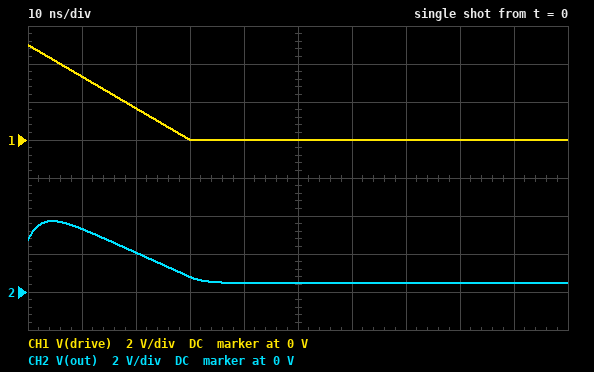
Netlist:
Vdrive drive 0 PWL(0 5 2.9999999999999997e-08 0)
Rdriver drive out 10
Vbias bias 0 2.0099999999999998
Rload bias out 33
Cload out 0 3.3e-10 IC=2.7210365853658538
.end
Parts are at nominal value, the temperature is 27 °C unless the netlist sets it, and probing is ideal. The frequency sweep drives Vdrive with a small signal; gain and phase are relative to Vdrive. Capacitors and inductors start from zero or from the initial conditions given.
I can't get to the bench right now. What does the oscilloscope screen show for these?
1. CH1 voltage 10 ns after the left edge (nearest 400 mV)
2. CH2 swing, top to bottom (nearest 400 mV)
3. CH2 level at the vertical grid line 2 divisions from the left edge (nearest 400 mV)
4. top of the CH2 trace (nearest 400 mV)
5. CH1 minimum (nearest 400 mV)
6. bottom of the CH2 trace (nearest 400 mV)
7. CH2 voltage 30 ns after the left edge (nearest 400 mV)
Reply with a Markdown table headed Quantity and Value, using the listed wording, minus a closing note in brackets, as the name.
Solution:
| Quantity | Value |
|---|---|
| CH1 voltage 10 ns after the left edge | 3.2 V |
| CH2 swing, top to bottom | 3.2 V |
| CH2 level at the vertical grid line 2 divisions from the left edge | 2.0 V |
| top of the CH2 trace | 3.6 V |
| CH1 minimum | 0 V |
| bottom of the CH2 trace | 400 mV |
| CH2 voltage 30 ns after the left edge | 800 mV |
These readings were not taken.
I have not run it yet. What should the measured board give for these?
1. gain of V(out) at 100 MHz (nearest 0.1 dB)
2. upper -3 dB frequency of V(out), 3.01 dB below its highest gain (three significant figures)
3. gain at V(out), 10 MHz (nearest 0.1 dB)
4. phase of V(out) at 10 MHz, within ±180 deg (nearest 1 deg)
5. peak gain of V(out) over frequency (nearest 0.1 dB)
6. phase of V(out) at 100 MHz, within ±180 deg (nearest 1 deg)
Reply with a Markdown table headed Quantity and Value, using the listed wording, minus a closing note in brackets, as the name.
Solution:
| Quantity | Value |
|---|---|
| gain of V(out) at 100 MHz | -7.8 dB |
| upper -3 dB frequency of V(out), 3.01 dB below its highest gain | 62.8 MHz |
| gain at V(out), 10 MHz | -2.4 dB |
| phase of V(out) at 10 MHz, within ±180 deg | -9 deg |
| peak gain of V(out) over frequency | -2.3 dB |
| phase of V(out) at 100 MHz, within ±180 deg | -58 deg |
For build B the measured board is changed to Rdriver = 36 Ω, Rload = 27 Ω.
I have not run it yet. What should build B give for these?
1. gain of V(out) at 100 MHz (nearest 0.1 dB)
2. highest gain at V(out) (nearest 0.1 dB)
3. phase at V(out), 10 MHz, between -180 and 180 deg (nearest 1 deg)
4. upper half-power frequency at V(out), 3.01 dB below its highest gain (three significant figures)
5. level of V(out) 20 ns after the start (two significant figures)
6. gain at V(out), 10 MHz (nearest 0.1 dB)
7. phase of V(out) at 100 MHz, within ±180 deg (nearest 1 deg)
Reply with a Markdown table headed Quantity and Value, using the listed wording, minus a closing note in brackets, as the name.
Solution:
| Quantity | Value |
|---|---|
| gain of V(out) at 100 MHz | -17.9 dB |
| highest gain at V(out) | -7.4 dB |
| phase at V(out), 10 MHz, between -180 and 180 deg | -18 deg |
| upper half-power frequency at V(out), 3.01 dB below its highest gain | 31.3 MHz |
| level of V(out) 20 ns after the start | 2.2 V |
| gain at V(out), 10 MHz | -7.8 dB |
| phase of V(out) at 100 MHz, within ±180 deg | -73 deg |
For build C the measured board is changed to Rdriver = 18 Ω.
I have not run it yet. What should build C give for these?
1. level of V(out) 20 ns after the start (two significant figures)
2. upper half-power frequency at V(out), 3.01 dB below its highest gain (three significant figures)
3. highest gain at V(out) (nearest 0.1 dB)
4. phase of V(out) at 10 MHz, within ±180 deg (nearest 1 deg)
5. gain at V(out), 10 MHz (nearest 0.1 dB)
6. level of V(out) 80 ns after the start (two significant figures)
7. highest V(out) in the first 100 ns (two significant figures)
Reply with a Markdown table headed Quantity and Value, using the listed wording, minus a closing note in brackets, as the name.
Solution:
| Quantity | Value |
|---|---|
| level of V(out) 20 ns after the start | 2.2 V |
| upper half-power frequency at V(out), 3.01 dB below its highest gain | 41.4 MHz |
| highest gain at V(out) | -3.8 dB |
| phase of V(out) at 10 MHz, within ±180 deg | -14 deg |
| gain at V(out), 10 MHz | -4.0 dB |
| level of V(out) 80 ns after the start | 710 mV |
| highest V(out) in the first 100 ns | 3.4 V |
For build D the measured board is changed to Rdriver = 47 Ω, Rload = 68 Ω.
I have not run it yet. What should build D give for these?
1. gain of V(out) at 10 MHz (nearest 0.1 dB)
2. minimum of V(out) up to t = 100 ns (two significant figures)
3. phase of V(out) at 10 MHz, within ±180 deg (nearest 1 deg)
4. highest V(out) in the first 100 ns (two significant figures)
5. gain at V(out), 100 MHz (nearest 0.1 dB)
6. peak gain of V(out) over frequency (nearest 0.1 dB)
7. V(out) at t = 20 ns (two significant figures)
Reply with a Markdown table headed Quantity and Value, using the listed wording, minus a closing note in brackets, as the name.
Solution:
| Quantity | Value |
|---|---|
| gain of V(out) at 10 MHz | -5.8 dB |
| minimum of V(out) up to t = 100 ns | 820 mV |
| phase of V(out) at 10 MHz, within ±180 deg | -30 deg |
| highest V(out) in the first 100 ns | 3.1 V |
| gain at V(out), 100 MHz | -19.9 dB |
| peak gain of V(out) over frequency | -4.6 dB |
| V(out) at t = 20 ns | 2.5 V |
